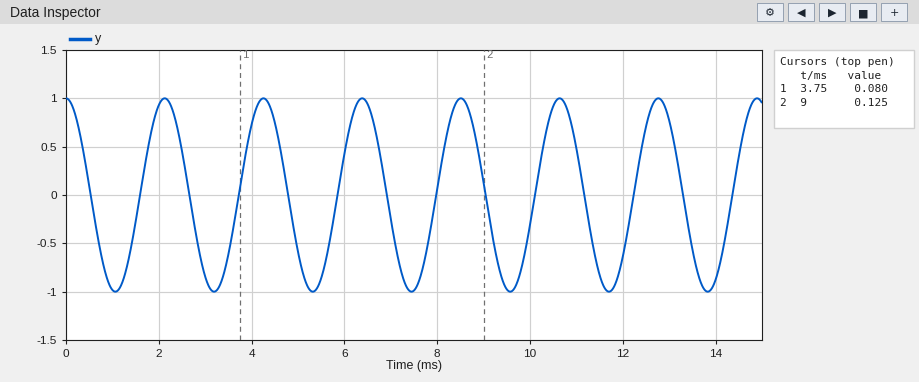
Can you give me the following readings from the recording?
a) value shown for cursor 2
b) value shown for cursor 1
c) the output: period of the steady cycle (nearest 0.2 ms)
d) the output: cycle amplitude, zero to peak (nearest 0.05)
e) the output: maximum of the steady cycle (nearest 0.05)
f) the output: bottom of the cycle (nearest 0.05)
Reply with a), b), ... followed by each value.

a) 0.125
b) 0.080
c) 2.2 ms
d) 1.00
e) 1.00
f) -1.00
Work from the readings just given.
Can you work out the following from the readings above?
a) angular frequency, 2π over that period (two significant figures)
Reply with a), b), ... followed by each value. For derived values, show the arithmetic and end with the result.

a) 2π / 2.2 = 2.9 rad/ms
